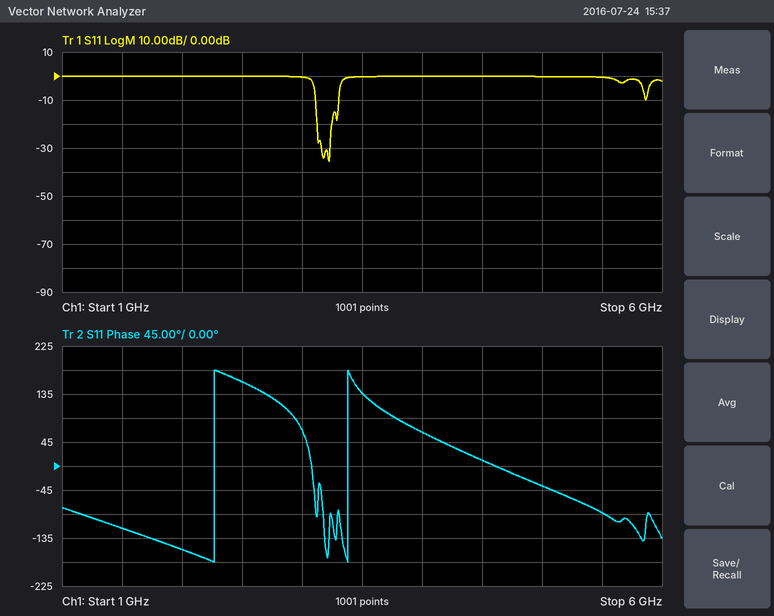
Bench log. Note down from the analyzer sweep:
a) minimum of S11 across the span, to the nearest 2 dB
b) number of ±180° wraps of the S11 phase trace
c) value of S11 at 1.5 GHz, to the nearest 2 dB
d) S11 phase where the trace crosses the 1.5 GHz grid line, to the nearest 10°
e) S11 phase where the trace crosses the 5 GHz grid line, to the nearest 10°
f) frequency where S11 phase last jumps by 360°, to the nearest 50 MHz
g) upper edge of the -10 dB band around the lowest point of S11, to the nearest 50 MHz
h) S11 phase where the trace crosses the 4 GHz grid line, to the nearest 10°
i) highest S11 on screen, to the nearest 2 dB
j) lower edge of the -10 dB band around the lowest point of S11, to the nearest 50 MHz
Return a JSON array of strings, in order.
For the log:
["-36 dB", "2", "0 dB", "-120°", "-40°", "3.40 GHz", "3.30 GHz", "60°", "0 dB", "3.10 GHz"]
